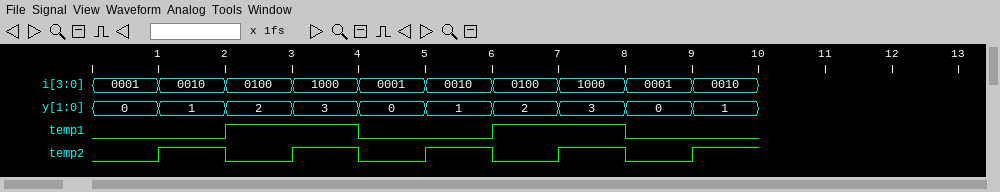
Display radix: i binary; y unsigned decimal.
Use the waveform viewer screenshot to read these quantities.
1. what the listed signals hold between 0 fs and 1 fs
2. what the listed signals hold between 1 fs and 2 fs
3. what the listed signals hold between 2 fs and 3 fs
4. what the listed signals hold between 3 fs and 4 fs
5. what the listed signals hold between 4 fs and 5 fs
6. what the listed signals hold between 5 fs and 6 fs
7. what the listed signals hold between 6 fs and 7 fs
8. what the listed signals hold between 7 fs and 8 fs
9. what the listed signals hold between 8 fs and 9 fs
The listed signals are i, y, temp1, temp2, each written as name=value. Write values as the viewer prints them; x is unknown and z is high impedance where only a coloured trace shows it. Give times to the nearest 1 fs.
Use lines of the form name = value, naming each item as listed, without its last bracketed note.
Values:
what the listed signals hold between 0 fs and 1 fs = i=0001, y=0, temp1=0, temp2=0
what the listed signals hold between 1 fs and 2 fs = i=0010, y=1, temp1=0, temp2=1
what the listed signals hold between 2 fs and 3 fs = i=0100, y=2, temp1=1, temp2=0
what the listed signals hold between 3 fs and 4 fs = i=1000, y=3, temp1=1, temp2=1
what the listed signals hold between 4 fs and 5 fs = i=0001, y=0, temp1=0, temp2=0
what the listed signals hold between 5 fs and 6 fs = i=0010, y=1, temp1=0, temp2=1
what the listed signals hold between 6 fs and 7 fs = i=0100, y=2, temp1=1, temp2=0
what the listed signals hold between 7 fs and 8 fs = i=1000, y=3, temp1=1, temp2=1
what the listed signals hold between 8 fs and 9 fs = i=0001, y=0, temp1=0, temp2=0
